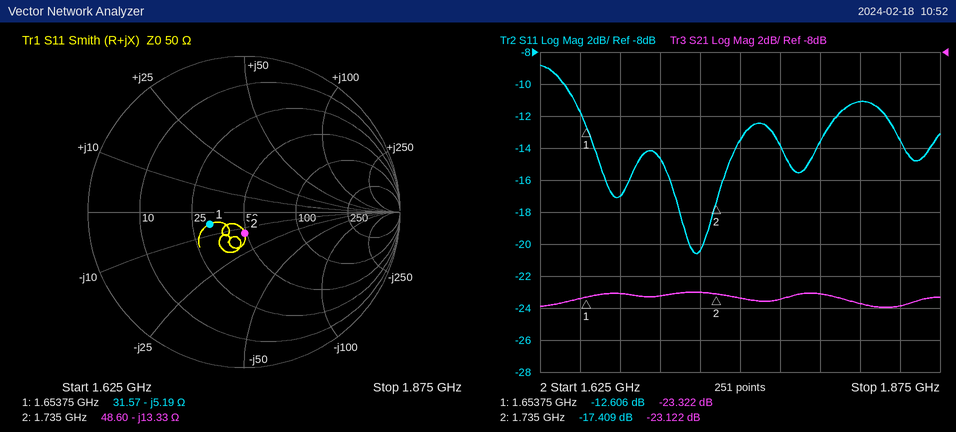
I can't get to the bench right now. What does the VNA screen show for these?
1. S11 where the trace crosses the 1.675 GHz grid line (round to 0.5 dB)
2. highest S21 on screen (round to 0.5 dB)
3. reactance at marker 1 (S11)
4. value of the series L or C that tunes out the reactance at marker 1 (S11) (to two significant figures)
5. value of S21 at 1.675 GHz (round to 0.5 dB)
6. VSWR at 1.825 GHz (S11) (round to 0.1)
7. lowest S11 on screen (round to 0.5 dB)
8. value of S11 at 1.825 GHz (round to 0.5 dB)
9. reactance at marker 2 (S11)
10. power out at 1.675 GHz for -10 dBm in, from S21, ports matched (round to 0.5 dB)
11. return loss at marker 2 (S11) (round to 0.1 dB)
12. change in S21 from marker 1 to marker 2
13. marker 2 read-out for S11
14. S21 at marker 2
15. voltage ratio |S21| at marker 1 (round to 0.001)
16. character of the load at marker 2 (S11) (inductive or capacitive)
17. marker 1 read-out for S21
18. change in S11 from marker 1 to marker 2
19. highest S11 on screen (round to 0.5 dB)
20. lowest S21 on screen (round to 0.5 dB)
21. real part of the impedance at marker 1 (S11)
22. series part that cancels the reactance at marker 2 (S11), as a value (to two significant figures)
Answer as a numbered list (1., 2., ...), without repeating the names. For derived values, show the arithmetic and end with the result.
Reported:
1. -17.0 dB
2. -23.0 dB
3. -5.19 Ω
4. L = 5.19 Ω/(2π × 1.65375 GHz) ≈ 499 pH, so 500 pH to two significant figures
5. -23.0 dB
6. |Γ| = 10^(-11/20) = 0.2818; VSWR = (1 + 0.2818)/(1 − 0.2818) ≈ 1.8
7. -20.5 dB
8. -11.0 dB
9. -13.33 Ω
10. -10 dBm + (-23.0 dB) = -33.0 dBm
11. 17.4 dB
12. -23.122 − (-23.322) = 0.200 dB
13. -17.409 dB
14. -23.122 dB
15. 10^(-23.322/20) ≈ 0.068
16. capacitive
17. -23.322 dB
18. -17.409 − (-12.606) = -4.803 dB
19. -9.0 dB
20. -24.0 dB
21. 31.57 Ω
22. L = 13.33 Ω/(2π × 1.735 GHz) ≈ 1.2 nH
